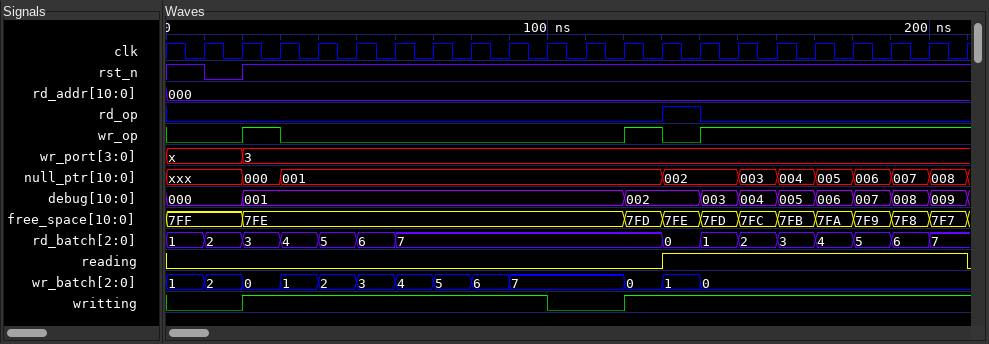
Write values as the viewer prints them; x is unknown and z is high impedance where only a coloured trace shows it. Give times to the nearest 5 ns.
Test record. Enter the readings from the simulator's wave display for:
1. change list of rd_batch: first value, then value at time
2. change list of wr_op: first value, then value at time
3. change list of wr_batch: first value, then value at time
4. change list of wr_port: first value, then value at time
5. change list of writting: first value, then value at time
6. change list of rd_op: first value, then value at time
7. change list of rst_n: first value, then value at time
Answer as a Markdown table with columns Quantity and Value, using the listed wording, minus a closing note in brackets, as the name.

| Quantity | Value |
|---|---|
| change list of rd_batch: first value, then value at time | 1, 2 at 10 ns, 3 at 20 ns, 4 at 30 ns, 5 at 40 ns, 6 at 50 ns, 7 at 60 ns, 0 at 130 ns, 1 at 140 ns, 2 at 150 ns, 3 at 160 ns, 4 at 170 ns, 5 at 180 ns, 6 at 190 ns, 7 at 200 ns |
| change list of wr_op: first value, then value at time | 0, 1 at 20 ns, 0 at 30 ns, 1 at 120 ns, 0 at 130 ns, 1 at 140 ns |
| change list of wr_batch: first value, then value at time | 1, 2 at 10 ns, 0 at 20 ns, 1 at 30 ns, 2 at 40 ns, 3 at 50 ns, 4 at 60 ns, 5 at 70 ns, 6 at 80 ns, 7 at 90 ns, 0 at 120 ns, 1 at 130 ns, 0 at 140 ns |
| change list of wr_port: first value, then value at time | x, 3 at 20 ns |
| change list of writting: first value, then value at time | 0, 1 at 20 ns, 0 at 100 ns, 1 at 120 ns |
| change list of rd_op: first value, then value at time | 0, 1 at 130 ns, 0 at 140 ns |
| change list of rst_n: first value, then value at time | 1, 0 at 10 ns, 1 at 20 ns |
